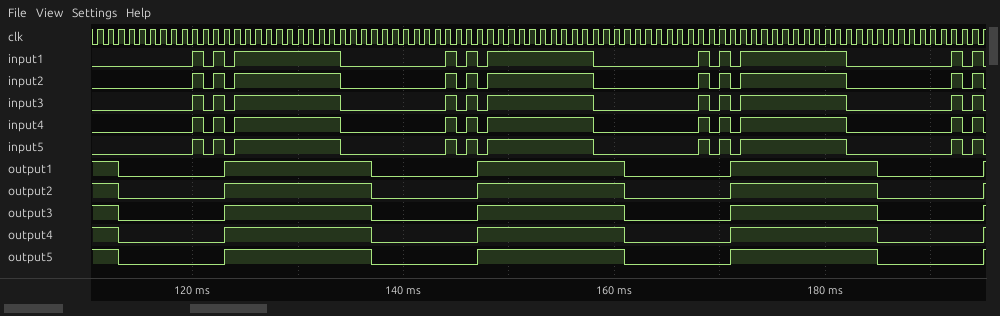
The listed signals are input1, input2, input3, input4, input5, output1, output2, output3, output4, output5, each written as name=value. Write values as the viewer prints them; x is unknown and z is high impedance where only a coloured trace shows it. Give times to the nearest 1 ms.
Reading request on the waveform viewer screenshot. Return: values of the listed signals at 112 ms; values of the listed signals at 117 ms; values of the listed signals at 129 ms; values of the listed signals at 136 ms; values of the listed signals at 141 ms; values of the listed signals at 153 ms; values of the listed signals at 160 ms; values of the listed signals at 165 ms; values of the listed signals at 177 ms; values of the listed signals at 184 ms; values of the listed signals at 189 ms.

input1=0, input2=0, input3=0, input4=0, input5=0, output1=1, output2=1, output3=1, output4=1, output5=1
input1=0, input2=0, input3=0, input4=0, input5=0, output1=0, output2=0, output3=0, output4=0, output5=0
input1=1, input2=1, input3=1, input4=1, input5=1, output1=1, output2=1, output3=1, output4=1, output5=1
input1=0, input2=0, input3=0, input4=0, input5=0, output1=1, output2=1, output3=1, output4=1, output5=1
input1=0, input2=0, input3=0, input4=0, input5=0, output1=0, output2=0, output3=0, output4=0, output5=0
input1=1, input2=1, input3=1, input4=1, input5=1, output1=1, output2=1, output3=1, output4=1, output5=1
input1=0, input2=0, input3=0, input4=0, input5=0, output1=1, output2=1, output3=1, output4=1, output5=1
input1=0, input2=0, input3=0, input4=0, input5=0, output1=0, output2=0, output3=0, output4=0, output5=0
input1=1, input2=1, input3=1, input4=1, input5=1, output1=1, output2=1, output3=1, output4=1, output5=1
input1=0, input2=0, input3=0, input4=0, input5=0, output1=1, output2=1, output3=1, output4=1, output5=1
input1=0, input2=0, input3=0, input4=0, input5=0, output1=0, output2=0, output3=0, output4=0, output5=0
